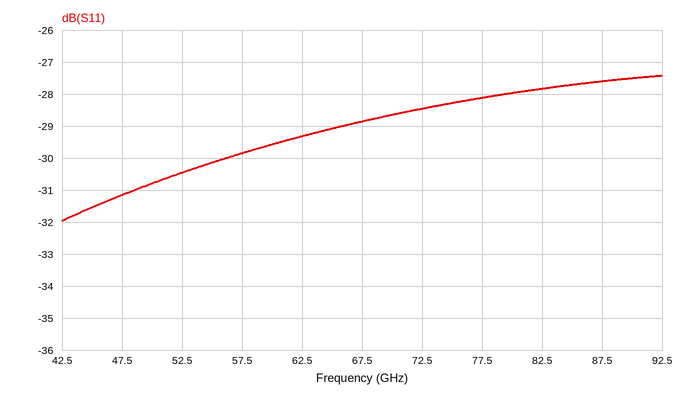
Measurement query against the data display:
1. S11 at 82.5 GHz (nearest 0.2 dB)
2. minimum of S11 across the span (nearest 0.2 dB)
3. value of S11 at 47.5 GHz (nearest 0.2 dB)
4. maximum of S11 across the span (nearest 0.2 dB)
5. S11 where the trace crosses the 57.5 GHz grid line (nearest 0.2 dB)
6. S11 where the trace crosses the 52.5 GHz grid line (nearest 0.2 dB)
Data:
-27.8 dB
-32.0 dB
-31.2 dB
-27.4 dB
-29.8 dB
-30.4 dB
